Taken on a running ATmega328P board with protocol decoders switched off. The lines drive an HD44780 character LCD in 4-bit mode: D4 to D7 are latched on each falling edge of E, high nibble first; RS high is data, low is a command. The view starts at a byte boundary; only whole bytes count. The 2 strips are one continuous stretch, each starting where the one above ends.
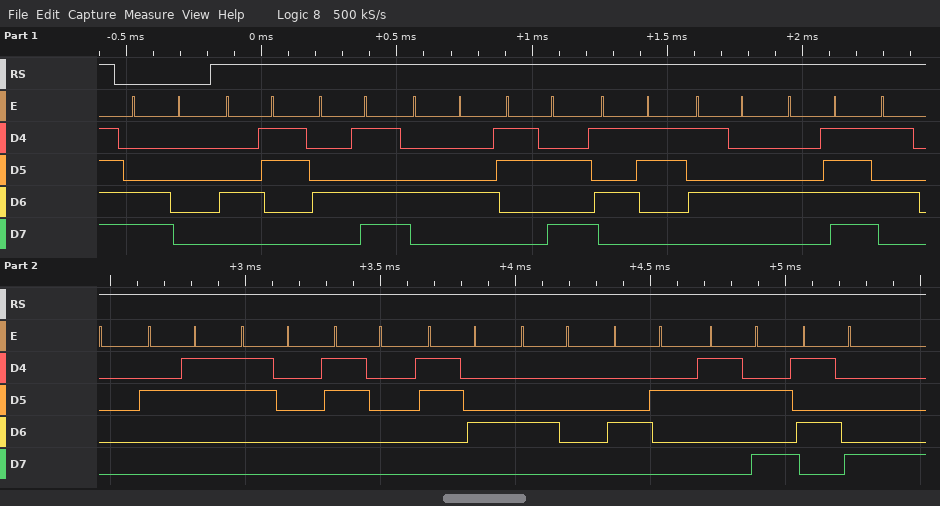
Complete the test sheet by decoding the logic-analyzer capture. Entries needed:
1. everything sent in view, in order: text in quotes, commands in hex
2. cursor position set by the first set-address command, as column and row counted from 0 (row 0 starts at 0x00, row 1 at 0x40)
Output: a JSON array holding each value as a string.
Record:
["0xC0 \"CMD:STOP#004@B:X\"", "column 0, row 1"]
